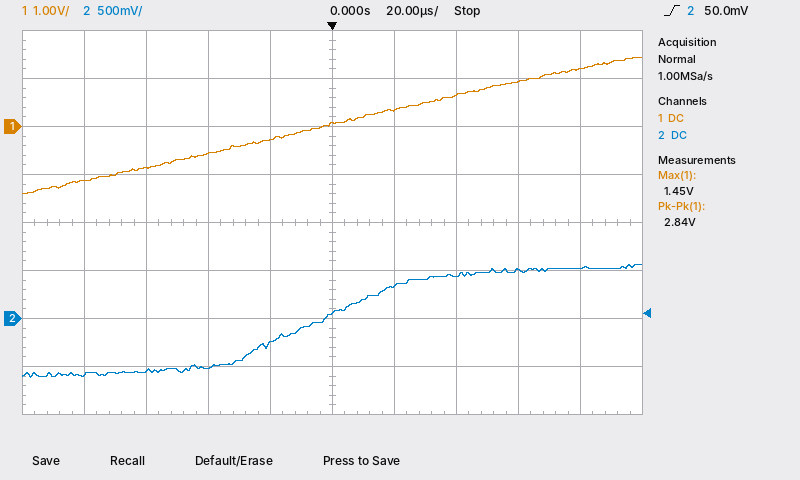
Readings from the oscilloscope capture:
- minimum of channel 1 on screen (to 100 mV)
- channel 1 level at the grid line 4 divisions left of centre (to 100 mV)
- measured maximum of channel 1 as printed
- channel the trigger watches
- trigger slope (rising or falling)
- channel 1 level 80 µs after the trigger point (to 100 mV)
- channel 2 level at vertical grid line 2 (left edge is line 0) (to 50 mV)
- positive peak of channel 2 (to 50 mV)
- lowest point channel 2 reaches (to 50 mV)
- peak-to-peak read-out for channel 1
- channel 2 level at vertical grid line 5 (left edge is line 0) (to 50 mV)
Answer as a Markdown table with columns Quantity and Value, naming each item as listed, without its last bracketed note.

| Quantity | Value |
|---|---|
| minimum of channel 1 on screen | -1.4 V |
| channel 1 level at the grid line 4 divisions left of centre | -1.1 V |
| measured maximum of channel 1 as printed | 1.45 V |
| channel the trigger watches | channel 2 |
| trigger slope | rising |
| channel 1 level 80 µs after the trigger point | 1.2 V |
| channel 2 level at vertical grid line 2 (left edge is line 0) | -550 mV |
| positive peak of channel 2 | 550 mV |
| lowest point channel 2 reaches | -600 mV |
| peak-to-peak read-out for channel 1 | 2.84 V |
| channel 2 level at vertical grid line 5 (left edge is line 0) | 50 mV |
